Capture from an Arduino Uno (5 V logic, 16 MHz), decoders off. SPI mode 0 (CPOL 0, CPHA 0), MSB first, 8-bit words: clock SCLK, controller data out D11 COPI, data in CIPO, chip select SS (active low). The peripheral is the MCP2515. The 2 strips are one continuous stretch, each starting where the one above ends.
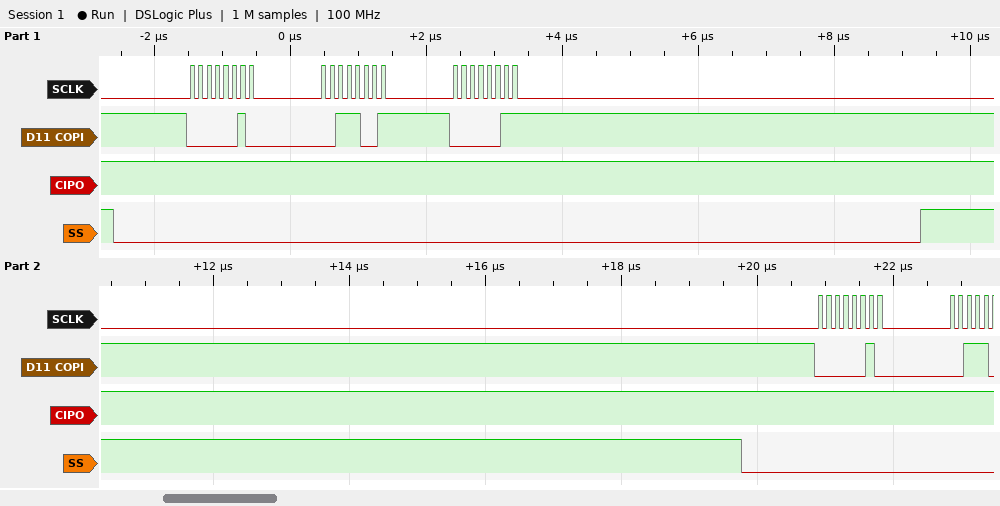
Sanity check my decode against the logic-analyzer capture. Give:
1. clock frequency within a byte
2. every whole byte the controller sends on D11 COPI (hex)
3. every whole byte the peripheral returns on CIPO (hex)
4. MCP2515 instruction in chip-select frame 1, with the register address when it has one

8 MHz
02 39 03 02
FF FF FF FF
WRITE 0x39
